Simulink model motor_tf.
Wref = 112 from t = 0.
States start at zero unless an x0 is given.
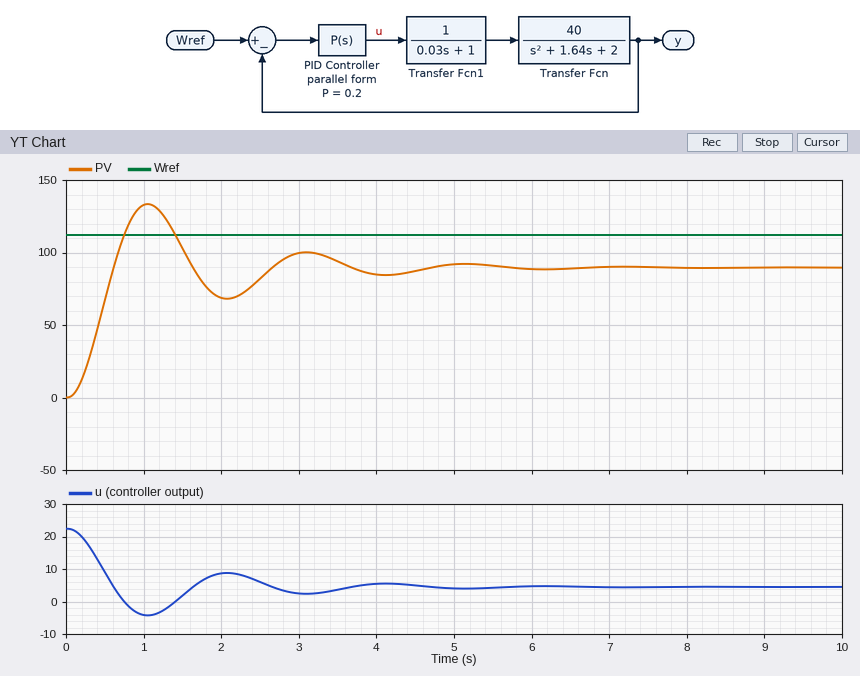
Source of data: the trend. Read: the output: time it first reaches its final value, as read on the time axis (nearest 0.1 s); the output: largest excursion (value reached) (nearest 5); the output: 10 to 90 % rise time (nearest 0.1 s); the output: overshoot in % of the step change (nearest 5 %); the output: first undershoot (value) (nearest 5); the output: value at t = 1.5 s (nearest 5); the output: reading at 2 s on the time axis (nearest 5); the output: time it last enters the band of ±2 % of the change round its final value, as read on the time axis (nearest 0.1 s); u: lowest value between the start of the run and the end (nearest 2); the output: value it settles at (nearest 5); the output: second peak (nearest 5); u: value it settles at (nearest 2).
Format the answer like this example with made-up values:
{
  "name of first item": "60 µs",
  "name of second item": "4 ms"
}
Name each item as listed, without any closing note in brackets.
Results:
{
  "the output: time it first reaches its final value, as read on the time axis": "0.6 s",
  "the output: largest excursion (value reached)": "135",
  "the output: 10 to 90 % rise time": "0.4 s",
  "the output: overshoot in % of the step change": "50 %",
  "the output: first undershoot (value)": "70",
  "the output: value at t = 1.5 s": "105",
  "the output: reading at 2 s on the time axis": "70",
  "the output: time it last enters the band of ±2 % of the change round its final value, as read on the time axis": "5.4 s",
  "u: lowest value between the start of the run and the end": "-4",
  "the output: value it settles at": "90",
  "the output: second peak": "100",
  "u: value it settles at": "4"
}
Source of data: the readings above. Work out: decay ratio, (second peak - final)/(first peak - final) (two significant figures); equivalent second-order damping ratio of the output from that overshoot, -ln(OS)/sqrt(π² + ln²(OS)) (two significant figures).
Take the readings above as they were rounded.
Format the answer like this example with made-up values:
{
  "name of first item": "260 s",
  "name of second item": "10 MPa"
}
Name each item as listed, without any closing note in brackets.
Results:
{
  "decay ratio, (second peak - final)/(first peak - final)": "0.22",
  "equivalent second-order damping ratio of the output from that overshoot, -ln(OS)/sqrt(π² + ln²(OS))": "0.22"
}
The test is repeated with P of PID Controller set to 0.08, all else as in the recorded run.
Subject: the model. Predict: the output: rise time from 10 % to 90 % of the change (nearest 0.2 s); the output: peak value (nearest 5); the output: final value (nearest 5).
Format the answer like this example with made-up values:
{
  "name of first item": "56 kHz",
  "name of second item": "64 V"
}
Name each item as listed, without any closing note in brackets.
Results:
{
  "the output: rise time from 10 % to 90 % of the change": "0.6 s",
  "the output: peak value": "90",
  "the output: final value": "70"
}
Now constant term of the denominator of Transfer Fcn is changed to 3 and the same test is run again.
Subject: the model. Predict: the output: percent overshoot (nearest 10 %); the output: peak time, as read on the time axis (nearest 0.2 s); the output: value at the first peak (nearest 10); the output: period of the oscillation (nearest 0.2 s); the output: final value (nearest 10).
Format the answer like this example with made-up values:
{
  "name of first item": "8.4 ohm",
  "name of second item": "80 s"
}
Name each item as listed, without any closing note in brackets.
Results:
{
  "the output: percent overshoot": "50 %",
  "the output: peak time, as read on the time axis": "1.0 s",
  "the output: value at the first peak": "120",
  "the output: period of the oscillation": "2.0 s",
  "the output: final value": "80"
}
